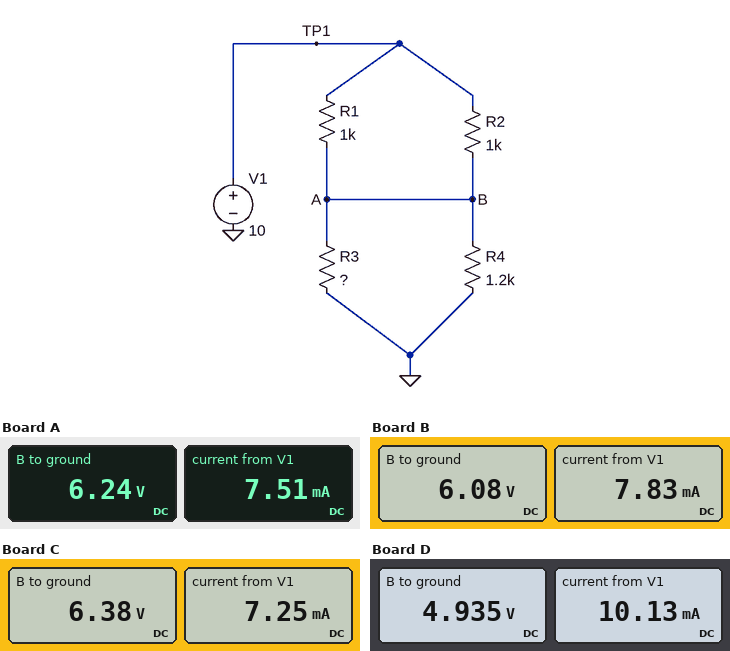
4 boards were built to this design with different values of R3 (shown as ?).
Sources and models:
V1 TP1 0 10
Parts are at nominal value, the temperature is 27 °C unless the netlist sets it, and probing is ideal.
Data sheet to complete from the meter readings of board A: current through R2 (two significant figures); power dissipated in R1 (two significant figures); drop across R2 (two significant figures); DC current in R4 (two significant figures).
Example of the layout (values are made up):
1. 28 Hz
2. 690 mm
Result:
1. 3.8 mA
2. 14 mW
3. 3.8 V
4. 5.2 mA
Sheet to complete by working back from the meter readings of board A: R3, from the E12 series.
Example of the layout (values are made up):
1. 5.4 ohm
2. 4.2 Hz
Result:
1. 2.7 kΩ
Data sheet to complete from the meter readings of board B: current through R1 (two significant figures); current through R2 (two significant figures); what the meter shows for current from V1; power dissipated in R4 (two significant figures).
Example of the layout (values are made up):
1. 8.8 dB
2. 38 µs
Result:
1. 3.9 mA
2. 3.9 mA
3. 7.83 mA
4. 31 mW
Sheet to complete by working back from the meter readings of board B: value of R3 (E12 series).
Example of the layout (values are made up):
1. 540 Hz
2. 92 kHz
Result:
1. 2.2 kΩ
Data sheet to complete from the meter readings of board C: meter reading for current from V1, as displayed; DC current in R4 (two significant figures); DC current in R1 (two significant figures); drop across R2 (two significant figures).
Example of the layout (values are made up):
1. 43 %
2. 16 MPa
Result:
1. 7.25 mA
2. 5.3 mA
3. 3.6 mA
4. 3.6 V
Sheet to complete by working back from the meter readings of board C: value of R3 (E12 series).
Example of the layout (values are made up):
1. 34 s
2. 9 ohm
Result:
1. 3.3 kΩ
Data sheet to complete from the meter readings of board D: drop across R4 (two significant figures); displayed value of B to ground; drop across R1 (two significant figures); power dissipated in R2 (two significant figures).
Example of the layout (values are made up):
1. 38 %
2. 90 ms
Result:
1. 4.9 V
2. 4.935 V
3. 5.1 V
4. 26 mW
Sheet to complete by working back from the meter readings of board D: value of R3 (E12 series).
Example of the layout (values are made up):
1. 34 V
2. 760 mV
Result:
1. 820 Ω
